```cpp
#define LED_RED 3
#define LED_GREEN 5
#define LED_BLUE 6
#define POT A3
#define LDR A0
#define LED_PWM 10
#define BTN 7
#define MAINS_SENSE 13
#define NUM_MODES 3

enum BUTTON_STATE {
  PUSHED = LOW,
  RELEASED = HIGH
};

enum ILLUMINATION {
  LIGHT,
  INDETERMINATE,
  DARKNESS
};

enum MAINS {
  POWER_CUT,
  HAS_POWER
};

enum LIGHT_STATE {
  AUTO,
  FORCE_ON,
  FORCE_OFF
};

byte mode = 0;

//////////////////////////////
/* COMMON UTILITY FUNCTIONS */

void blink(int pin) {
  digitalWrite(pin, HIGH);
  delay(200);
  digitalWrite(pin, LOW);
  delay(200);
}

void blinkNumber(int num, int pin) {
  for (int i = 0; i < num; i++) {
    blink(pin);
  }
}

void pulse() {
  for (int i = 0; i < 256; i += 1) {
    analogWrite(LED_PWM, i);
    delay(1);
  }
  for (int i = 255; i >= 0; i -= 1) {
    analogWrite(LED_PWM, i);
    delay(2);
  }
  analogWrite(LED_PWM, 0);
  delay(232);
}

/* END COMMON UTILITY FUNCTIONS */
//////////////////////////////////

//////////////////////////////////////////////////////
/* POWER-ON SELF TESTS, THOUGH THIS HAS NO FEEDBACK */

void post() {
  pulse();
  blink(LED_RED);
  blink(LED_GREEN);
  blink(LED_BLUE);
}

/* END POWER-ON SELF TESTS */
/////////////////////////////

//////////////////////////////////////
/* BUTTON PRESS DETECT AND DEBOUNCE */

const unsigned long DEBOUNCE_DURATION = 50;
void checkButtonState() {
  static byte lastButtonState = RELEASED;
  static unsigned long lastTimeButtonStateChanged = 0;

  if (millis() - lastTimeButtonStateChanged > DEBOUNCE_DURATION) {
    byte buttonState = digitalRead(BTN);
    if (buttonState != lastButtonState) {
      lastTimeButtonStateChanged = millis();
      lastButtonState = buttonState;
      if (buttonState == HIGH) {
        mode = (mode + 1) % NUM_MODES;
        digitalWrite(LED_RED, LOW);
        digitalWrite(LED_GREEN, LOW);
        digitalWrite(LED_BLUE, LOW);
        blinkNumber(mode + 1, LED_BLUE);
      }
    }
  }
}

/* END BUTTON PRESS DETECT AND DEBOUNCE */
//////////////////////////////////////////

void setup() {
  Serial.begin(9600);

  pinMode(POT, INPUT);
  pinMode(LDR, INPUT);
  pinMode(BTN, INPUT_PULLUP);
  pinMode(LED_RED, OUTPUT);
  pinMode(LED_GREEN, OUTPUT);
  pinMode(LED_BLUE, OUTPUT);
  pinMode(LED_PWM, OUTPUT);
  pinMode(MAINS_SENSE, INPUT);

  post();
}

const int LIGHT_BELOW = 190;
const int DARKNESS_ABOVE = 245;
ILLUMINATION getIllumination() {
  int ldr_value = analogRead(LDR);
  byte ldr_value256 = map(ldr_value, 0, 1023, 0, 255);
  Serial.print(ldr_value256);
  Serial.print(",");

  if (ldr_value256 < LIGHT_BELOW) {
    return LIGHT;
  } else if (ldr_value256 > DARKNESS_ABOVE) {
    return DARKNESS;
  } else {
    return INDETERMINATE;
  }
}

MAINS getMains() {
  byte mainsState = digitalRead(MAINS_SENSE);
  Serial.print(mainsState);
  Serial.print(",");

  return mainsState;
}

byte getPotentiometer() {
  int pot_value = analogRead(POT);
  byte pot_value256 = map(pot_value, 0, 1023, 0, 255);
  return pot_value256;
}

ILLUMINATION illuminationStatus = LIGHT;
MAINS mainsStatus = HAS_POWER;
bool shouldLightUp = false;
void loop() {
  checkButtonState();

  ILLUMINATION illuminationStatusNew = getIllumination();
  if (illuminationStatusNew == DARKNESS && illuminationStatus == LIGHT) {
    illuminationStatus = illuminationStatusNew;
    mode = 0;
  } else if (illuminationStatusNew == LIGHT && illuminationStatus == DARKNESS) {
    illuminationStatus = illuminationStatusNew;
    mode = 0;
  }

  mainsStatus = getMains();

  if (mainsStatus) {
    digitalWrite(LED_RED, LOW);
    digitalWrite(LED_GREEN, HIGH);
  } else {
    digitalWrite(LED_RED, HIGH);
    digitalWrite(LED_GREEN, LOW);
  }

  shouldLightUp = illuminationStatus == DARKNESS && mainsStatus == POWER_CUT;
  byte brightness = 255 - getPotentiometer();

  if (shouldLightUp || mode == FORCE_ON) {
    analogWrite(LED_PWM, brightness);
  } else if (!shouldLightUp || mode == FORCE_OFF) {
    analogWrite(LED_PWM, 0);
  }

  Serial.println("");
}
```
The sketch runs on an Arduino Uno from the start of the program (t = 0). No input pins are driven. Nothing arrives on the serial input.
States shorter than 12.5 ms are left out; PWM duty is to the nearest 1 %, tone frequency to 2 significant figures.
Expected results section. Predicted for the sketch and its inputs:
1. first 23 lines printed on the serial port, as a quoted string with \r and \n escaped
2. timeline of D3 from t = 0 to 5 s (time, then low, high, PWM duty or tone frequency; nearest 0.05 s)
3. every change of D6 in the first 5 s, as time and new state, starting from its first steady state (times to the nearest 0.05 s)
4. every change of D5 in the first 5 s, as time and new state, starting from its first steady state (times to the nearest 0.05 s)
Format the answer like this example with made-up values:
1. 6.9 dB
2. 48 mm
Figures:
1. "0,0,\r\n0,0,\r\n0,0,\r\n0,0,\r\n0,0,\r\n0,0,\r\n0,0,\r\n0,0,\r\n0,0,\r\n0,0,\r\n0,0,\r\n0,0,\r\n0,0,\r\n0,0,\r\n0,0,\r\n0,0,\r\n0,0,\r\n0,0,\r\n0,0,\r\n0,0,\r\n0,0,\r\n0,0,\r\n0,0,\r\n"
2. 0 s low; 1 s high; 1.2 s low; 2.2 s high
3. 0 s low; 1.8 s high; 2 s low
4. 0 s low; 1.4 s high; 1.6 s low
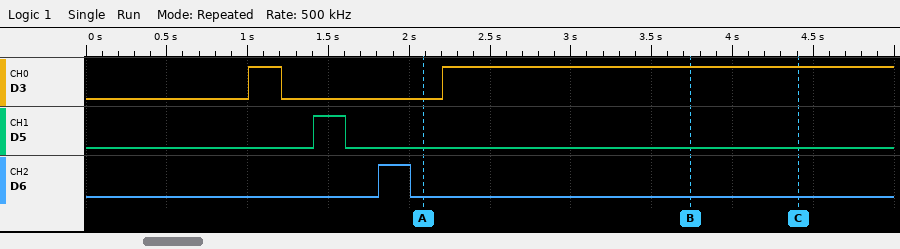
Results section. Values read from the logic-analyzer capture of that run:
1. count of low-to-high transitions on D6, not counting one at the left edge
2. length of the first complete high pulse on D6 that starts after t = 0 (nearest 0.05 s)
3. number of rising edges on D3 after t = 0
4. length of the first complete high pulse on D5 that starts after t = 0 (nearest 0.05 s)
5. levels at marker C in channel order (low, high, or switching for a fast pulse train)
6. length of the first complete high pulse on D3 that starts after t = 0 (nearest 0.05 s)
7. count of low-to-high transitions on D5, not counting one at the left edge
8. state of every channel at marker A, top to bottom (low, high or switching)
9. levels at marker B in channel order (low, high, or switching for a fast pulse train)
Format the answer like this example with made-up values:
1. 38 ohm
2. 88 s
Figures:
1. 1
2. 0.20 s
3. 2
4. 0.20 s
5. D3 high, D5 low, D6 low
6. 0.20 s
7. 1
8. D3 low, D5 low, D6 low
9. D3 high, D5 low, D6 low
